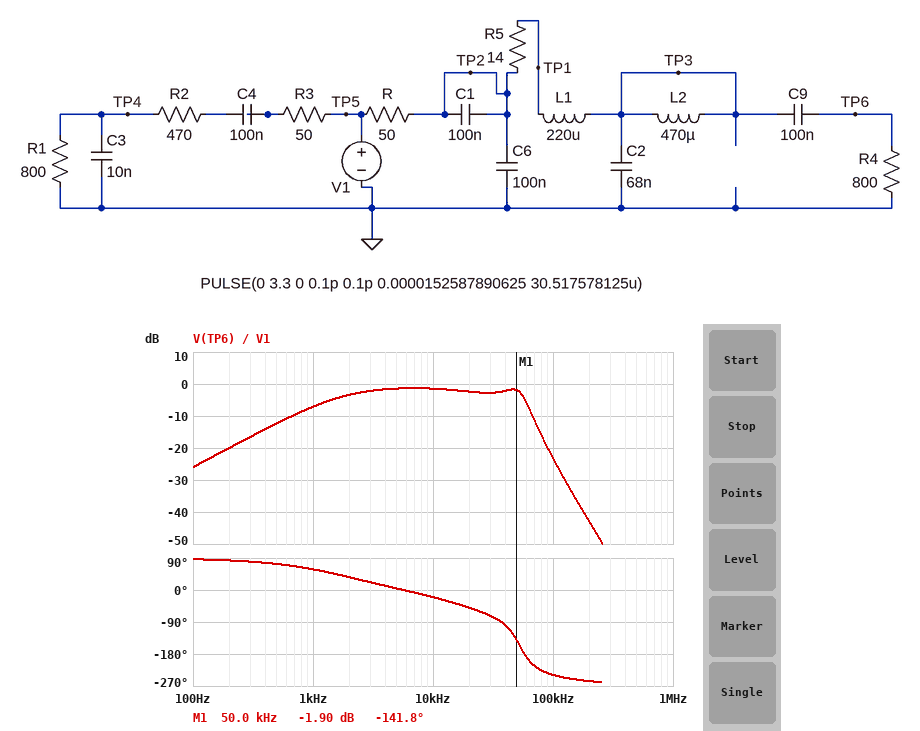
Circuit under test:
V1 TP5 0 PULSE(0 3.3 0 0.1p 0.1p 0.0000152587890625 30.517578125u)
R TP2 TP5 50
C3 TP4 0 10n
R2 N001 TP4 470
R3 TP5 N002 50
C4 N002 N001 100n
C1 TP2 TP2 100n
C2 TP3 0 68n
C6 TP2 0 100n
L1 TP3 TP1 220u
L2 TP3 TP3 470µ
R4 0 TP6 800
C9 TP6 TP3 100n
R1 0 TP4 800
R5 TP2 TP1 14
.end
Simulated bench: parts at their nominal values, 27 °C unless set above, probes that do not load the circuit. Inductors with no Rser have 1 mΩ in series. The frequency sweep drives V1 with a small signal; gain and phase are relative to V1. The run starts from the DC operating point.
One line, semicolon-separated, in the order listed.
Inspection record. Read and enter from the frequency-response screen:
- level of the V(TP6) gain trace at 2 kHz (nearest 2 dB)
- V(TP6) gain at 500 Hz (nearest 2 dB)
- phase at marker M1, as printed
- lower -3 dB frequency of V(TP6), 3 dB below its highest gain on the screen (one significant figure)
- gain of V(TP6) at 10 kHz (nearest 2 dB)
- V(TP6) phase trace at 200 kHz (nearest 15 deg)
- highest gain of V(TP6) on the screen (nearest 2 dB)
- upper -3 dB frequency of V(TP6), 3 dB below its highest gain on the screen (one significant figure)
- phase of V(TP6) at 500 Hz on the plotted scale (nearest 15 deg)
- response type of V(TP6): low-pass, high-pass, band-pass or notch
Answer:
-4 dB; -12 dB; -141.8 deg; 2 kHz; -2 dB; -255 deg; -2 dB; 60 kHz; 75 deg; band-pass
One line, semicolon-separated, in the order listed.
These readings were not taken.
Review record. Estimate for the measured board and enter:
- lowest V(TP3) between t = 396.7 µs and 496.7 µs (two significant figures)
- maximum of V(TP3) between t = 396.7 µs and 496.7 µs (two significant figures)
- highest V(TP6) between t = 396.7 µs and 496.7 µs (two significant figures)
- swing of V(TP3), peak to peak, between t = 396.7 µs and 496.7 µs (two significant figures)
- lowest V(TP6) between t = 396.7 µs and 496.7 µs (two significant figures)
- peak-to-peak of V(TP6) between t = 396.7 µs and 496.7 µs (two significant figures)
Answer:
160 mV; 3.1 V; 1.5 V; 3.0 V; -1.5 V; 3.0 V
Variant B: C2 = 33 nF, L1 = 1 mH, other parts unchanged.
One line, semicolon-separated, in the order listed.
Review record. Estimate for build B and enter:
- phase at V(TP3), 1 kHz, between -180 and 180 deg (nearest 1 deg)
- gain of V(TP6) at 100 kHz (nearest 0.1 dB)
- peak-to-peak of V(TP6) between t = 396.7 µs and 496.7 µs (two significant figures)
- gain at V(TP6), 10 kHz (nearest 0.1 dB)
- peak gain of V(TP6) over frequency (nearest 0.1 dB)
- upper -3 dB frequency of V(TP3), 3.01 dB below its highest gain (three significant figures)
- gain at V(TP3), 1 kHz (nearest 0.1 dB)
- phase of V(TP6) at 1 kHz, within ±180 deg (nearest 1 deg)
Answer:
-4 deg; -31.8 dB; 5.6 V; -0.4 dB; 4.2 dB; 34.2 kHz; -0.1 dB; 59 deg
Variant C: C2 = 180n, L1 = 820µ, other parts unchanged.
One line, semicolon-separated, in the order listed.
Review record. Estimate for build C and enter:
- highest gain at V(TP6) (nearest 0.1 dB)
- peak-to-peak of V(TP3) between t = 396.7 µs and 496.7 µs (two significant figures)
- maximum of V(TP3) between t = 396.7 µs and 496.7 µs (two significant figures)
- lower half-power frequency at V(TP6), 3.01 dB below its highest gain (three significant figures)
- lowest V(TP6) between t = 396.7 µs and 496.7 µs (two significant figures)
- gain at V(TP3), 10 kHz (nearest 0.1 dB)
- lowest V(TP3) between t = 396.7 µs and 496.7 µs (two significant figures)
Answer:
-0.3 dB; 630 mV; 2.0 V; 2.00 kHz; -310 mV; -0.2 dB; 1.3 V
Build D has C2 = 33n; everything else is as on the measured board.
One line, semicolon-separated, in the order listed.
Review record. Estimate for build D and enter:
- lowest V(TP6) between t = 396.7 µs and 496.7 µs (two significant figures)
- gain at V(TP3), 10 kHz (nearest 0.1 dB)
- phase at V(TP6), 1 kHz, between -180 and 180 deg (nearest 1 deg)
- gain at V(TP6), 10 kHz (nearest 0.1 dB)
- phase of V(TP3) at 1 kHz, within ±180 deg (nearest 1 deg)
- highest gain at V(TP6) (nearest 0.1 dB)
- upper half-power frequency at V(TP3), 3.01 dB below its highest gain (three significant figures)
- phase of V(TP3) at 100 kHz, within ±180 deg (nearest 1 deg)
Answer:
-1.5 V; -1.1 dB; 59 deg; -1.3 dB; -4 deg; 0.5 dB; 74.4 kHz; 127 deg
